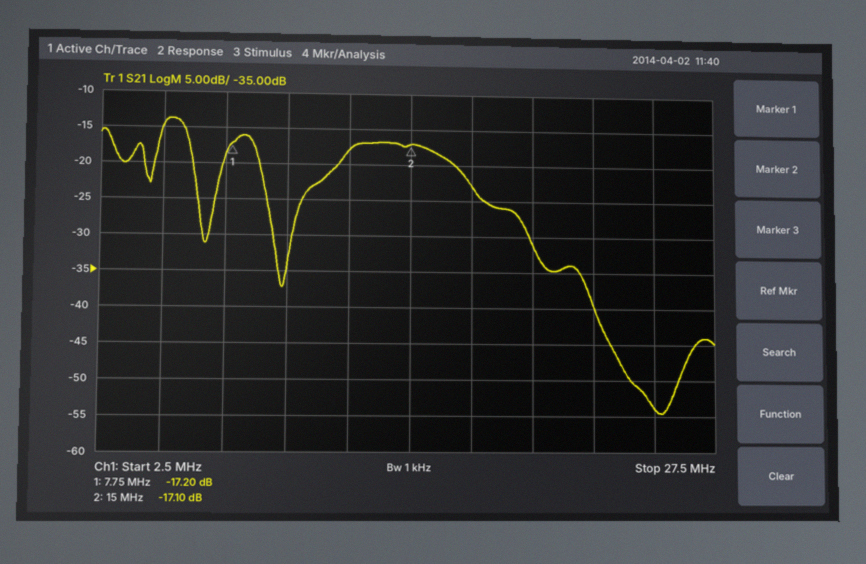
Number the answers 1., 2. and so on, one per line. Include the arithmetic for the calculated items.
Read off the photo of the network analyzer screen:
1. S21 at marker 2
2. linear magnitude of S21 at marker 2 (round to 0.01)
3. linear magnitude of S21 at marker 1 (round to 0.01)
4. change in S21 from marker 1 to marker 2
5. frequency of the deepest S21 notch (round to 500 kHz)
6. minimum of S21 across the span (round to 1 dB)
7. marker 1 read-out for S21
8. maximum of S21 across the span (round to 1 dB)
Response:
1. -17.10 dB
2. 10^(-17.1/20) ≈ 0.14
3. 10^(-17.2/20) ≈ 0.14
4. -17.1 − (-17.2) = 0.10 dB
5. 25.5 MHz
6. -55 dB
7. -17.20 dB
8. -14 dB
